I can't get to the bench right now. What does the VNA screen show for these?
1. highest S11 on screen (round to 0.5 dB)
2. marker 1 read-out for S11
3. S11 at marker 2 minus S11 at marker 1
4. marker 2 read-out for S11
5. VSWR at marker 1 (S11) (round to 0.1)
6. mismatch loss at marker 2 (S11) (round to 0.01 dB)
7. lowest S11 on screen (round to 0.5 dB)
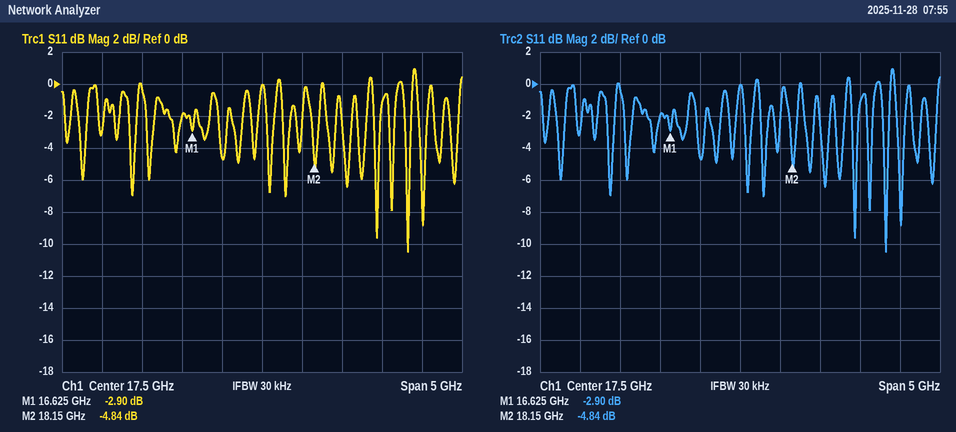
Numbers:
1.0 dB
-2.90 dB
-1.94 dB
-4.84 dB
6.0
1.73 dB
-10.5 dB
